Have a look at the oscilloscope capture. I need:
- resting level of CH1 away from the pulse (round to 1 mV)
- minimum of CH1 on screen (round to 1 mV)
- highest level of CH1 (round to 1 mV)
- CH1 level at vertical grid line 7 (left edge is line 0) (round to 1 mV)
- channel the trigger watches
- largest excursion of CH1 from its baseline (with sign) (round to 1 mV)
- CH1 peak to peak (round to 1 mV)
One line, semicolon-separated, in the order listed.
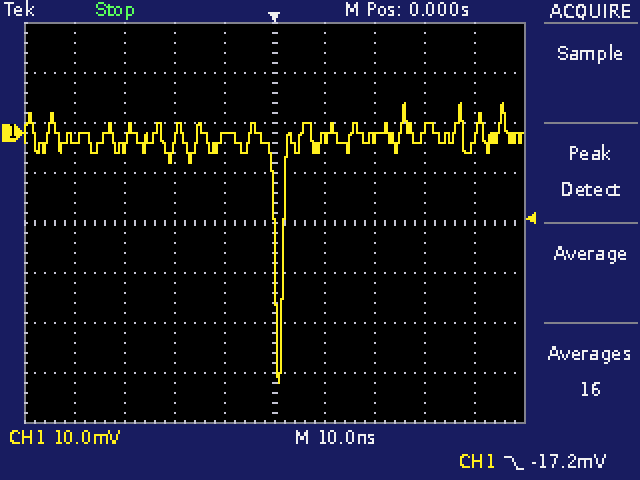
-1 mV; -50 mV; 6 mV; -1 mV; CH1; -49 mV; 56 mV
